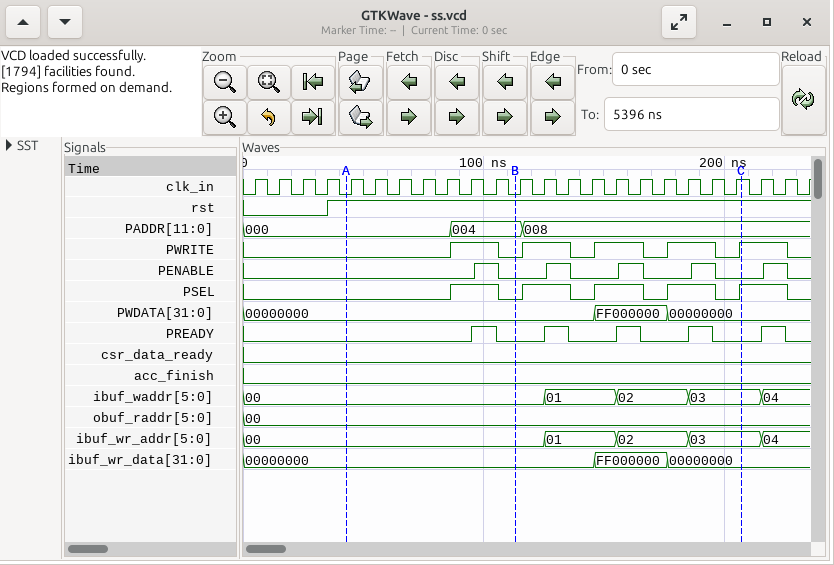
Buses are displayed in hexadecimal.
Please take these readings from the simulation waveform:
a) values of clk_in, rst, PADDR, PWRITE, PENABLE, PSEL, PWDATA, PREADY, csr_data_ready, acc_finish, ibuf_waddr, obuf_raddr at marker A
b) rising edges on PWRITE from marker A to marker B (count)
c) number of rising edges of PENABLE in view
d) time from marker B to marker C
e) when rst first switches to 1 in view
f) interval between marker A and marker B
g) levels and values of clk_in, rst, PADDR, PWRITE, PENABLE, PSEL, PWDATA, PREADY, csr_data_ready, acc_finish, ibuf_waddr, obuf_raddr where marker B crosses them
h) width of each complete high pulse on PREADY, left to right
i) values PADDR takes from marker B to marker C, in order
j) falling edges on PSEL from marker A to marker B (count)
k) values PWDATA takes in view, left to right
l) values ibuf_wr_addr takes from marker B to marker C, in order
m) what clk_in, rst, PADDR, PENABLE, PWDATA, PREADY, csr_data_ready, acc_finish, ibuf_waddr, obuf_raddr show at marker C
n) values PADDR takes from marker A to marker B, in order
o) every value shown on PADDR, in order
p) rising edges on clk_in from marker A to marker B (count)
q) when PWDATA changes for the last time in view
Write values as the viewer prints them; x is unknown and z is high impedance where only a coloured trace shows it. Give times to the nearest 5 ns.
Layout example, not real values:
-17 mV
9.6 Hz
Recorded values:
clk_in=0, rst=1, PADDR=000, PWRITE=0, PENABLE=0, PSEL=0, PWDATA=00000000, PREADY=0, csr_data_ready=0, acc_finish=0, ibuf_waddr=00, obuf_raddr=00
1
5
95 ns
35 ns
70 ns
clk_in=0, rst=1, PADDR=004, PWRITE=0, PENABLE=0, PSEL=0, PWDATA=00000000, PREADY=0, csr_data_ready=0, acc_finish=0, ibuf_waddr=00, obuf_raddr=00
10 ns, 10 ns, 10 ns, 10 ns, 10 ns
004, 008
1
00000000, FF000000, 00000000
00, 01, 02, 03
clk_in=1, rst=1, PADDR=008, PENABLE=0, PWDATA=00000000, PREADY=0, csr_data_ready=0, acc_finish=0, ibuf_waddr=03, obuf_raddr=00
000, 004
000, 004, 008
7
175 ns
